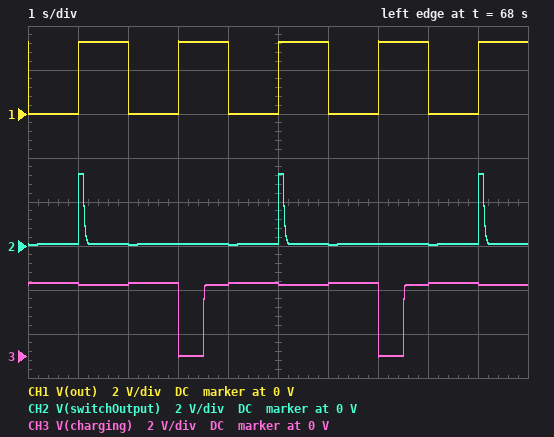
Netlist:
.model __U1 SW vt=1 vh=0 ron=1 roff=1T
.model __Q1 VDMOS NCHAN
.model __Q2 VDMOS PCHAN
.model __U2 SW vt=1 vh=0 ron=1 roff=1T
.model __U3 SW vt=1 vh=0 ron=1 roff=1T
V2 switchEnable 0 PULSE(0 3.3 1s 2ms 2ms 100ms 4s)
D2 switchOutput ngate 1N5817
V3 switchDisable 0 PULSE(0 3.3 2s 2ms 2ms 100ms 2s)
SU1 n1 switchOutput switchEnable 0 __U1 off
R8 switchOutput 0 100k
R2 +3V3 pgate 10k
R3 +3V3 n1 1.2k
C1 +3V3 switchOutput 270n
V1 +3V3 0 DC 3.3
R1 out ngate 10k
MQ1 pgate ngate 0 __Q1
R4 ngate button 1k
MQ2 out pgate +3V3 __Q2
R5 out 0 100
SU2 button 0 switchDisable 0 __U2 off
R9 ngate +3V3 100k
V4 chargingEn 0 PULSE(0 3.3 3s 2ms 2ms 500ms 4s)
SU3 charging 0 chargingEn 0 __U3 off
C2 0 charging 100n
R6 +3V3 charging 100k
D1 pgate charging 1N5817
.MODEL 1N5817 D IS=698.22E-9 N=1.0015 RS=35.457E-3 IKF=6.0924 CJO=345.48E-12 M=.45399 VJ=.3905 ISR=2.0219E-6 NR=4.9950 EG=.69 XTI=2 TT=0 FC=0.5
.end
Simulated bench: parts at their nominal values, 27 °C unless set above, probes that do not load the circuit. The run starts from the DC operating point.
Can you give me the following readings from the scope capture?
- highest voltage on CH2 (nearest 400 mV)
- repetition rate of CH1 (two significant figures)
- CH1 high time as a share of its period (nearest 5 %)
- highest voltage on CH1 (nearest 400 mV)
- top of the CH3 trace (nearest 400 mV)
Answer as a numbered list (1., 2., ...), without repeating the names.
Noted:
1. 3.2 V
2. 500 mHz
3. 50 %
4. 3.2 V
5. 3.2 V
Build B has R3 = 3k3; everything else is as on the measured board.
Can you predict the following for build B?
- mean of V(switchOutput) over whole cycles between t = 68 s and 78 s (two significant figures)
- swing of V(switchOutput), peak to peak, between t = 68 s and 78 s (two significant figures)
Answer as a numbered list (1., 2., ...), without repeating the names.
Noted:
1. 130 mV
2. 2.5 V
